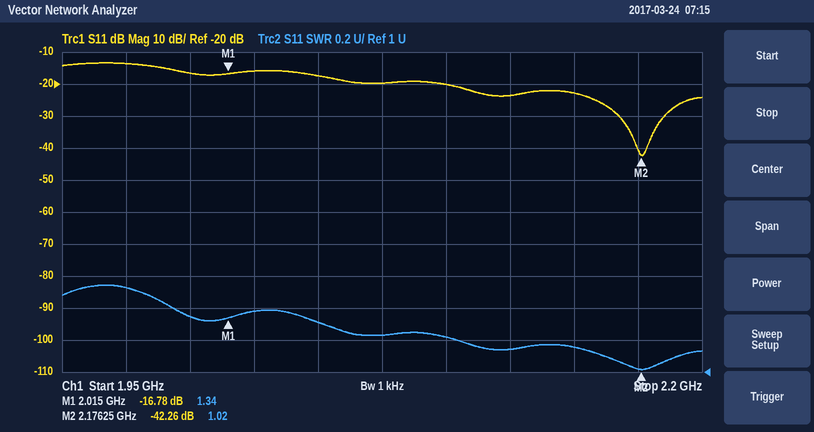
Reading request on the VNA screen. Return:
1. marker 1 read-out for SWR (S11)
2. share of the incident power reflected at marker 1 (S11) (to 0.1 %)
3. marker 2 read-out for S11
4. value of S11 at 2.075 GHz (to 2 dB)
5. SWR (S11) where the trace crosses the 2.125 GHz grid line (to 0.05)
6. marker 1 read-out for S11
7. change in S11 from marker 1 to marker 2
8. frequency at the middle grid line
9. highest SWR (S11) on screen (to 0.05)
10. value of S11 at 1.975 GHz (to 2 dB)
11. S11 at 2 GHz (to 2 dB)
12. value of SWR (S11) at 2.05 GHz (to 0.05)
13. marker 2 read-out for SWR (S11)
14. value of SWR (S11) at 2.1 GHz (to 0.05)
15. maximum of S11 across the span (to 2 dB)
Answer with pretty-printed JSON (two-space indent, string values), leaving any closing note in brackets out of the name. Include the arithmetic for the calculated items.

{
  "marker 1 read-out for SWR": "1.34",
  "share of the incident power reflected at marker 1 (S11)": "10^(-16.78/10) ≈ 2.1 %",
  "marker 2 read-out for S11": "-42.26 dB",
  "value of S11 at 2.075 GHz": "-20 dB",
  "SWR (S11) where the trace crosses the 2.125 GHz grid line": "1.15",
  "marker 1 read-out for S11": "-16.78 dB",
  "change in S11 from marker 1 to marker 2": "-42.26 − (-16.78) = -25.48 dB",
  "frequency at the middle grid line": "2.075 GHz",
  "highest SWR (S11) on screen": "1.55",
  "value of S11 at 1.975 GHz": "-14 dB",
  "S11 at 2 GHz": "-16 dB",
  "value of SWR (S11) at 2.05 GHz": "1.30",
  "marker 2 read-out for SWR": "1.02",
  "value of SWR (S11) at 2.1 GHz": "1.20",
  "maximum of S11 across the span": "-14 dB"
}
